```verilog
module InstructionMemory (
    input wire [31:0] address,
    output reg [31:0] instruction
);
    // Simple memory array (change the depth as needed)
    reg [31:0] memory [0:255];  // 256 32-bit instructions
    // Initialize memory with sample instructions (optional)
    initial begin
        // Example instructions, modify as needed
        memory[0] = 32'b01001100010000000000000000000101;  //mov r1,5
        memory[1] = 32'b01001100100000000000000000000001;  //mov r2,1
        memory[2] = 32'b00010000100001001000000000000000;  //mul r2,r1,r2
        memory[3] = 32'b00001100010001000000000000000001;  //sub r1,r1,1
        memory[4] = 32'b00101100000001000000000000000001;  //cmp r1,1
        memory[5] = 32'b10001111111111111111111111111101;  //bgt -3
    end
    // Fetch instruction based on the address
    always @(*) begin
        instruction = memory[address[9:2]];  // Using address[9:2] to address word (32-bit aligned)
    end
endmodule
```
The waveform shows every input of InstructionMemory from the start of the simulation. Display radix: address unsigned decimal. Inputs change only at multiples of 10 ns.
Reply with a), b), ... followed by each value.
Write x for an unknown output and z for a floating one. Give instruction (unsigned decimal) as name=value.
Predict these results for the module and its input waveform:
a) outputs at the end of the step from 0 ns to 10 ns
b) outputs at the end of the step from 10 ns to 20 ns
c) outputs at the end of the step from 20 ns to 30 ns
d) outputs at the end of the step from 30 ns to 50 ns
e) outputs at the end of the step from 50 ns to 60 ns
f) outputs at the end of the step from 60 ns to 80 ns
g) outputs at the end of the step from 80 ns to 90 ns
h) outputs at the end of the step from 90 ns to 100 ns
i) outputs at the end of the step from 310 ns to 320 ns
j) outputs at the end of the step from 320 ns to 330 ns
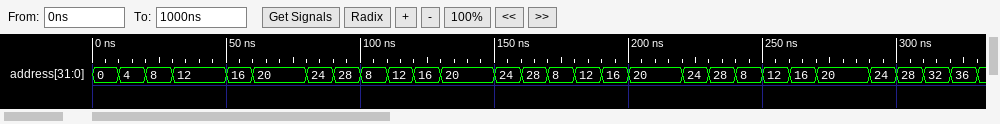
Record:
a) instruction=1279262725
b) instruction=1283457025
c) instruction=277118976
d) instruction=205783041
e) instruction=738459649
f) instruction=2415919101
g) instruction=x
h) instruction=x
i) instruction=x
j) instruction=x
